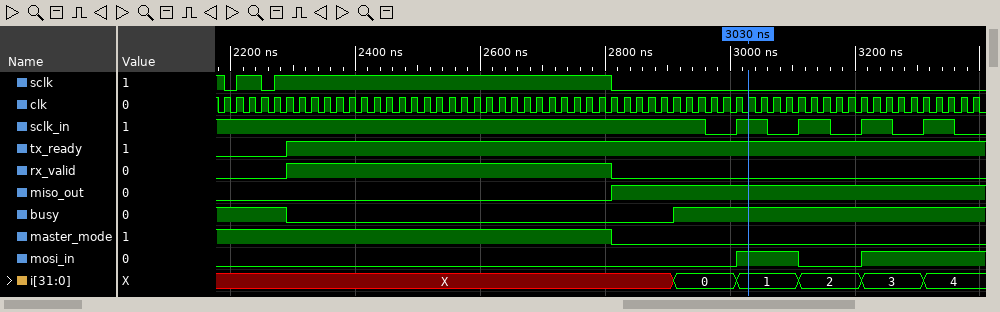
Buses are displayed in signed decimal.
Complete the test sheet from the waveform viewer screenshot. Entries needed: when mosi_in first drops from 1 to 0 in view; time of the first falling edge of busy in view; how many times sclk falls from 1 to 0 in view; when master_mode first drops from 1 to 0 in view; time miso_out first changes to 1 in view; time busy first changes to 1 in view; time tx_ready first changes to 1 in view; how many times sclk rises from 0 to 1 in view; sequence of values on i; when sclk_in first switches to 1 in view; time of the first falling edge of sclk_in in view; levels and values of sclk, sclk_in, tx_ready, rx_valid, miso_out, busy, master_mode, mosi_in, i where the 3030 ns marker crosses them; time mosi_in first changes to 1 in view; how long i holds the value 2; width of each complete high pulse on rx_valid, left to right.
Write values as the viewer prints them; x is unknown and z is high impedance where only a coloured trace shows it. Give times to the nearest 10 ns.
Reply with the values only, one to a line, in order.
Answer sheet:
3110 ns
2290 ns
3
2810 ns
2810 ns
2910 ns
2290 ns
2
X, 0, 1, 2, 3, 4
3010 ns
2960 ns
sclk=0, sclk_in=1, tx_ready=1, rx_valid=0, miso_out=1, busy=1, master_mode=0, mosi_in=1, i=1
3010 ns
100 ns
520 ns
